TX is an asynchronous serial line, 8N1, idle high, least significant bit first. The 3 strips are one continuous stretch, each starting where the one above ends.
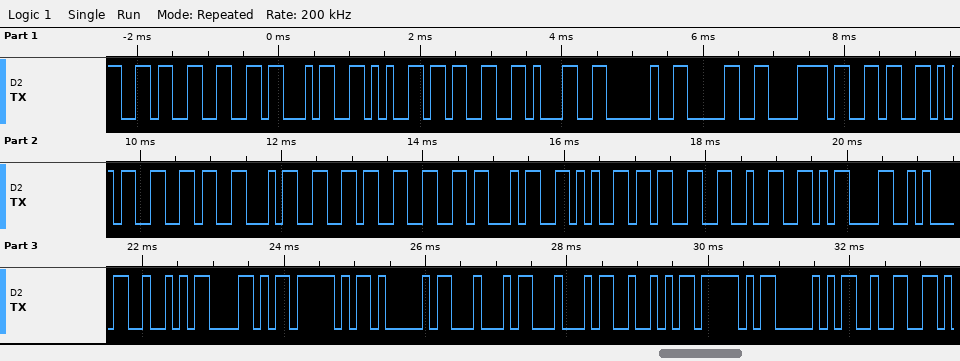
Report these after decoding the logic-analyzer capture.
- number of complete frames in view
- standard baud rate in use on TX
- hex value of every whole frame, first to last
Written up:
31
9600 baud
36 66 34 65 33 31 20 30 78 36 35 36 34 36 66 34 65 33 32 0D 0A 52 58 5F 41 44 44 52 5F 50 32
